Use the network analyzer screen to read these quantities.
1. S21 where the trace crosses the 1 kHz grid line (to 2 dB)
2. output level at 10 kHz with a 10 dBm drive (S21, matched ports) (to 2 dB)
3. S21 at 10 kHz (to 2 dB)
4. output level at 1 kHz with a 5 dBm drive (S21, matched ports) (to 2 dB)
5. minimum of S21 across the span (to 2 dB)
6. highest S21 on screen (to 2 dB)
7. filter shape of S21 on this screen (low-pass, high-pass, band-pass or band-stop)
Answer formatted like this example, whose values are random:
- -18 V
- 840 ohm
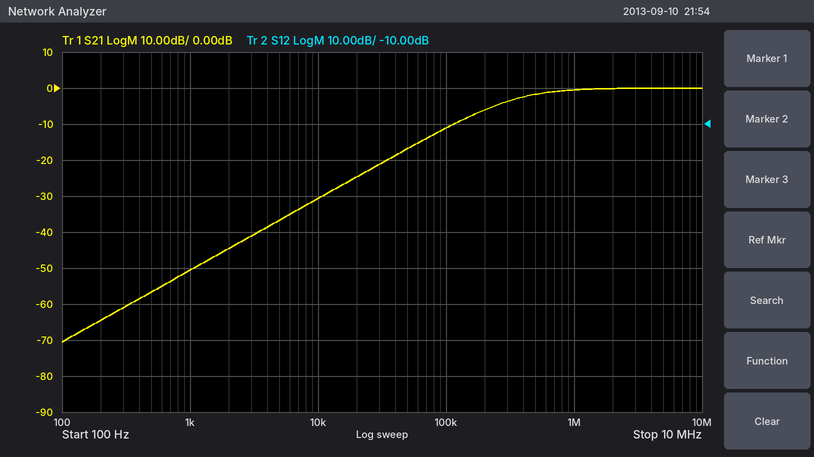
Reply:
- -50 dB
- -20 dBm
- -30 dB
- -46 dBm
- -70 dB
- 0 dB
- high-pass
